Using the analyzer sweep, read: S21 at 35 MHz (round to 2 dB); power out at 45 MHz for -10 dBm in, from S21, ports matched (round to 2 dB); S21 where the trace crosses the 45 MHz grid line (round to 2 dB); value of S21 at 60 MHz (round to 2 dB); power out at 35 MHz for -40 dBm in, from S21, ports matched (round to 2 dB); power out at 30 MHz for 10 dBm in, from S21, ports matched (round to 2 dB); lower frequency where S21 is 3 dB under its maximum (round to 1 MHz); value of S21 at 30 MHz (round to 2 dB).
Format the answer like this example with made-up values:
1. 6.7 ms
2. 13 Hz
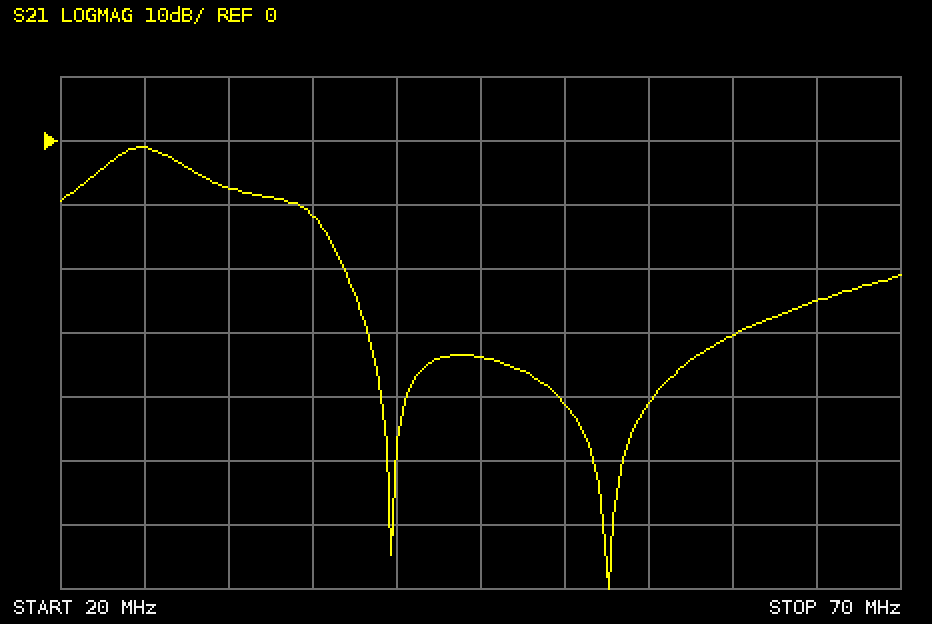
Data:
1. -12 dB
2. -44 dBm
3. -34 dB
4. -30 dB
5. -52 dBm
6. 2 dBm
7. 23 MHz
8. -8 dB
